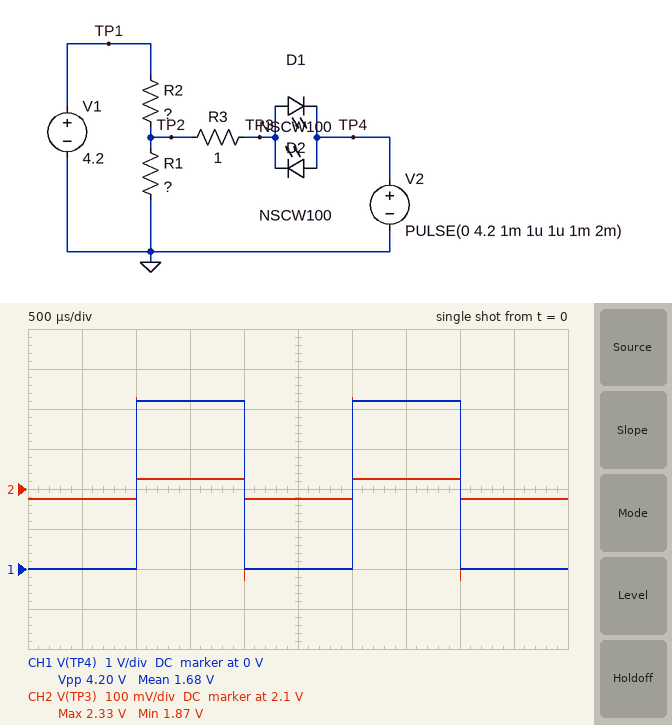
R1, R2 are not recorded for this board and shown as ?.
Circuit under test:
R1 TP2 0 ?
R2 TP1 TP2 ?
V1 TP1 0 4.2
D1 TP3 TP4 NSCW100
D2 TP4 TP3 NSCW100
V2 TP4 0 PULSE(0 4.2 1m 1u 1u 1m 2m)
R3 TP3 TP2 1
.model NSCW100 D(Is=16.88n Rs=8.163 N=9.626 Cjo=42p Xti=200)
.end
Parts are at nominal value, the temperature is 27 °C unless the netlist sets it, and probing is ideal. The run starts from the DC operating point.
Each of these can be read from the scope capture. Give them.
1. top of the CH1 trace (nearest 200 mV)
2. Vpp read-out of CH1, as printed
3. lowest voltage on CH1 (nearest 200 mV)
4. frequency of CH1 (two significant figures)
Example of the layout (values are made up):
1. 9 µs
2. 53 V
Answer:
1. 4.2 V
2. 4.20 V
3. 0 V
4. 500 Hz
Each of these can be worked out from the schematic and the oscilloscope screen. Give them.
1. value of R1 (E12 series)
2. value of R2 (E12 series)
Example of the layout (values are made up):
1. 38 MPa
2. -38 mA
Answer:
1. 680 Ω
2. 680 Ω
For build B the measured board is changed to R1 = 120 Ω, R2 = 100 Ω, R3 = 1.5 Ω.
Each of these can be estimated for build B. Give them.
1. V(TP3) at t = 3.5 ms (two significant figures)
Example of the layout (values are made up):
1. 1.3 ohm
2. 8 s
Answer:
1. 2.3 V
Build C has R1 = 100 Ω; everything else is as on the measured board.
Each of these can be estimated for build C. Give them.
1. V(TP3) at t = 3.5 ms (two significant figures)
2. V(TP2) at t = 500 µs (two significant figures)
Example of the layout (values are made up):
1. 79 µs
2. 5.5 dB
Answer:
1. 1.0 V
2. 540 mV
